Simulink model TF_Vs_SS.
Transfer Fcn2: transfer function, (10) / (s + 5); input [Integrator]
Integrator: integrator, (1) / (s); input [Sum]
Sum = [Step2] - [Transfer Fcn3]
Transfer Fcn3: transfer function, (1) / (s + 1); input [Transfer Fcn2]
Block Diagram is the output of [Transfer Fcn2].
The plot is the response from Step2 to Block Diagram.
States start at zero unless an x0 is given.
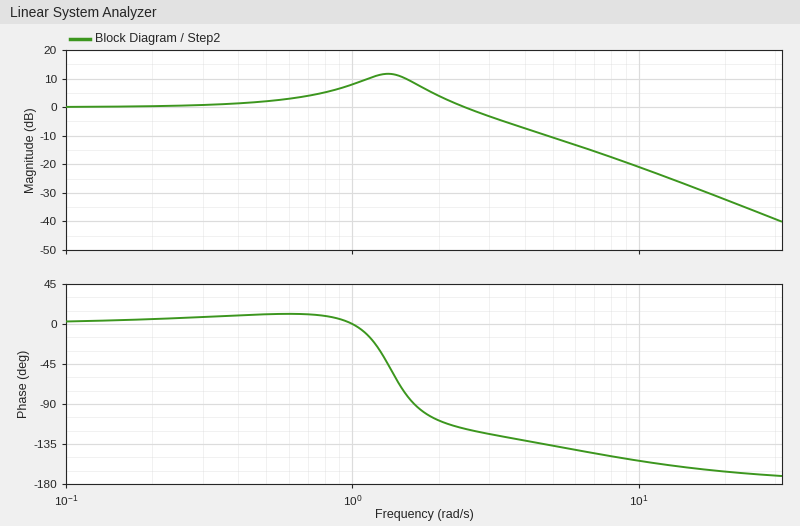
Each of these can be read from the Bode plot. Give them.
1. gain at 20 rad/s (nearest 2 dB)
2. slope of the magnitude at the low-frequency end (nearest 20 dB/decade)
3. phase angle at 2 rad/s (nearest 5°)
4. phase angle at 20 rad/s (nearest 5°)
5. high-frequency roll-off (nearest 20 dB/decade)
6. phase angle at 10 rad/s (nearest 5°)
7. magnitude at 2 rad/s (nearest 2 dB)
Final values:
-32 dB
0 dB/decade
-110°
-165°
-40 dB/decade
-155°
4 dB
